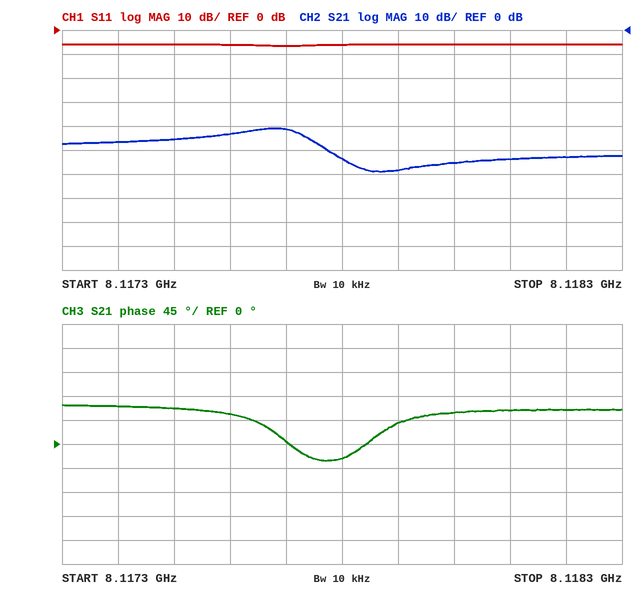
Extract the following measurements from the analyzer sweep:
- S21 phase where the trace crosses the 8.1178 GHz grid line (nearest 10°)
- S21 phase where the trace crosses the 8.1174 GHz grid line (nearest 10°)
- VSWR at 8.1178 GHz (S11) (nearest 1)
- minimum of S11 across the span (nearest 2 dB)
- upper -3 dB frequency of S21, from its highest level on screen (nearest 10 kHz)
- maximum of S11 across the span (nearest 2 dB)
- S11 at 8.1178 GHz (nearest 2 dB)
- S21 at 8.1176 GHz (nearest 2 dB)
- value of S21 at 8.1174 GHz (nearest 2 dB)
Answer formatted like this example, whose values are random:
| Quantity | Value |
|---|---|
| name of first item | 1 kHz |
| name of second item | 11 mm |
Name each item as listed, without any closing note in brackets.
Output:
| Quantity | Value |
|---|---|
| S21 phase where the trace crosses the 8.1178 GHz grid line | -30° |
| S21 phase where the trace crosses the 8.1174 GHz grid line | 70° |
| VSWR at 8.1178 GHz (S11) | 3 |
| minimum of S11 across the span | -6 dB |
| upper -3 dB frequency of S21, from its highest level on screen | 8.11773 GHz |
| maximum of S11 across the span | -6 dB |
| S11 at 8.1178 GHz | -6 dB |
| S21 at 8.1176 GHz | -44 dB |
| value of S21 at 8.1174 GHz | -46 dB |
